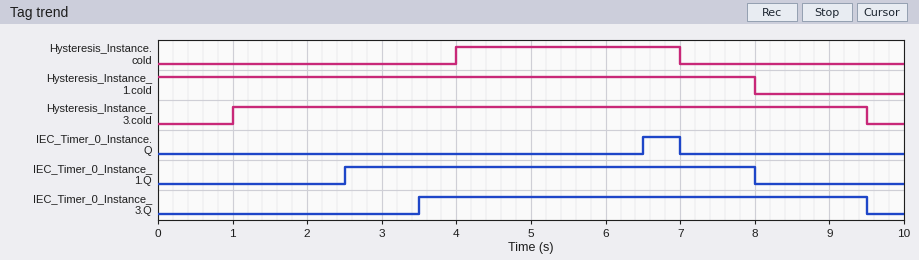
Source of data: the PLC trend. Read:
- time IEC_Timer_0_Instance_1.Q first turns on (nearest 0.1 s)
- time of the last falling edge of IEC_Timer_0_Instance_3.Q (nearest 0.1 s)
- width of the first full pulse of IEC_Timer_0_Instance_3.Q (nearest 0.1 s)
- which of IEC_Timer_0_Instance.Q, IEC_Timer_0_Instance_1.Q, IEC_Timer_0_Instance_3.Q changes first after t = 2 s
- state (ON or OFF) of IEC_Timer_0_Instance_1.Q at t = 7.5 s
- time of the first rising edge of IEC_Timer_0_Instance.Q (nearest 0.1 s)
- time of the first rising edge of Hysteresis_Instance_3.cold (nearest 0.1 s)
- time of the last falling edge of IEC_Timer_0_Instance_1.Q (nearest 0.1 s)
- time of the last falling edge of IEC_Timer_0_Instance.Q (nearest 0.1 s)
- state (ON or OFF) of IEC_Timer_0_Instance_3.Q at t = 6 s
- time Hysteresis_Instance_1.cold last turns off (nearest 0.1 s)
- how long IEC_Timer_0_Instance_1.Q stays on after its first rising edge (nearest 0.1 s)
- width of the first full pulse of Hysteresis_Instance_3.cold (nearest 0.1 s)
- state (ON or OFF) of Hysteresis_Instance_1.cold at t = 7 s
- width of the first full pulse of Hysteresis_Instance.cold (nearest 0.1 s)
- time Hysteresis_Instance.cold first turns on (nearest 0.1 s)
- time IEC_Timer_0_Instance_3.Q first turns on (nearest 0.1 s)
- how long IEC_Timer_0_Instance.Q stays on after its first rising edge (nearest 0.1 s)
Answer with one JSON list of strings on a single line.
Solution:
["2.5 s", "9.5 s", "6.0 s", "IEC_Timer_0_Instance_1.Q", "ON", "6.5 s", "1.0 s", "8.0 s", "7.0 s", "ON", "8.0 s", "5.5 s", "8.5 s", "ON", "3.0 s", "4.0 s", "3.5 s", "0.5 s"]
